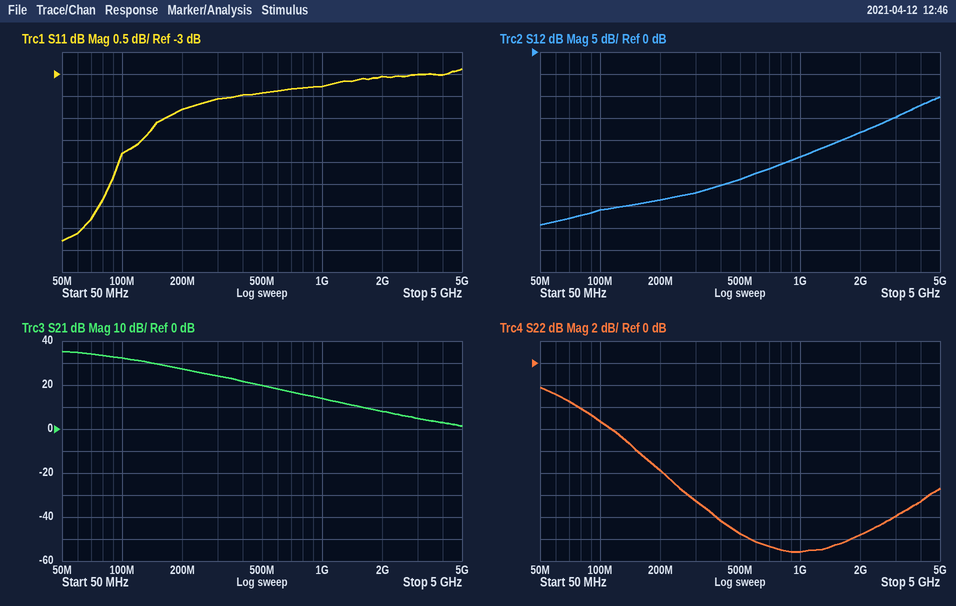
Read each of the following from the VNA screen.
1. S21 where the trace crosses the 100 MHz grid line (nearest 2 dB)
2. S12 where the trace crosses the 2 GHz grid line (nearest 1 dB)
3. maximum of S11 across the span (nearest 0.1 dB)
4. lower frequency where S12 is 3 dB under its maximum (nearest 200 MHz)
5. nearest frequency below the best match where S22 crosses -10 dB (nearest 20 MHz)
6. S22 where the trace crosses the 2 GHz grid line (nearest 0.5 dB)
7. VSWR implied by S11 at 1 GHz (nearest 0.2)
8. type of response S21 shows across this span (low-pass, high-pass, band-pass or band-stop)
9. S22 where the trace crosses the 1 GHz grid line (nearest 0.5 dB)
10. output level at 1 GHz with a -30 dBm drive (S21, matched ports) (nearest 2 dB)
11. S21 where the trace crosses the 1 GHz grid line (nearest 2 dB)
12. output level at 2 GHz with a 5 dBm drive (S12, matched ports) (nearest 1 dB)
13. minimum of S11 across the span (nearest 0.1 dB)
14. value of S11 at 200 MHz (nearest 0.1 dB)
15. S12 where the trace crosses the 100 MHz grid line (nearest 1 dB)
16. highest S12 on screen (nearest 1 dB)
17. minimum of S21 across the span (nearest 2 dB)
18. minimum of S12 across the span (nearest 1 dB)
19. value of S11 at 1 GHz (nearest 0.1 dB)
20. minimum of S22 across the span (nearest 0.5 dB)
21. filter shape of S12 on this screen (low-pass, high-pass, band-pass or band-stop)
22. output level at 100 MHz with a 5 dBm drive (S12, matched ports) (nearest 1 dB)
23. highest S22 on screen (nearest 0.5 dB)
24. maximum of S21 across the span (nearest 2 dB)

32 dB
-18 dB
-2.9 dB
3.6 GHz
200 MHz
-15.5 dB
5.4
low-pass
-17.0 dB
-16 dBm
14 dB
-13 dBm
-6.8 dB
-3.8 dB
-36 dB
-10 dB
2 dB
-39 dB
-3.3 dB
-17.0 dB
high-pass
-31 dBm
-2.0 dB
36 dB
